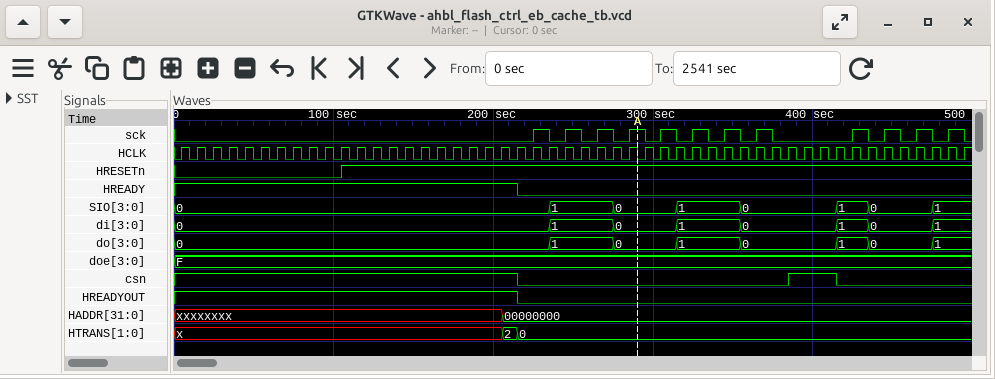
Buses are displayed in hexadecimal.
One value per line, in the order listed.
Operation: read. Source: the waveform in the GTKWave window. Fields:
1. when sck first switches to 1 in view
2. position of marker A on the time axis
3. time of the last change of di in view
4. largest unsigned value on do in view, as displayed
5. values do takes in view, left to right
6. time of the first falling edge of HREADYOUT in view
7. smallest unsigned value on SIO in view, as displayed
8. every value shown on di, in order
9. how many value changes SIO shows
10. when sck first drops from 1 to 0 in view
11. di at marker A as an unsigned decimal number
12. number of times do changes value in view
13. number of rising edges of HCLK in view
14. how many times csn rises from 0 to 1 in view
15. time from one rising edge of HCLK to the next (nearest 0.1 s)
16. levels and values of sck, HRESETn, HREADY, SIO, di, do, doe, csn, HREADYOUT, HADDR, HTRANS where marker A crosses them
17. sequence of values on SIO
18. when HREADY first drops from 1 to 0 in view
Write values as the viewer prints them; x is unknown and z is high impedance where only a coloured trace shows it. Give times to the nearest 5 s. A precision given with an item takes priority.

225 s
290 s
475 s
1
0, 1, 0, 1, 0, 1, 0, 1
215 s
0
0, 1, 0, 1, 0, 1, 0, 1
7
235 s
0
7
50
1
10 s
sck=1, HRESETn=1, HREADY=0, SIO=0, di=0, do=0, doe=F, csn=0, HREADYOUT=0, HADDR=00000000, HTRANS=0
0, 1, 0, 1, 0, 1, 0, 1
215 s
